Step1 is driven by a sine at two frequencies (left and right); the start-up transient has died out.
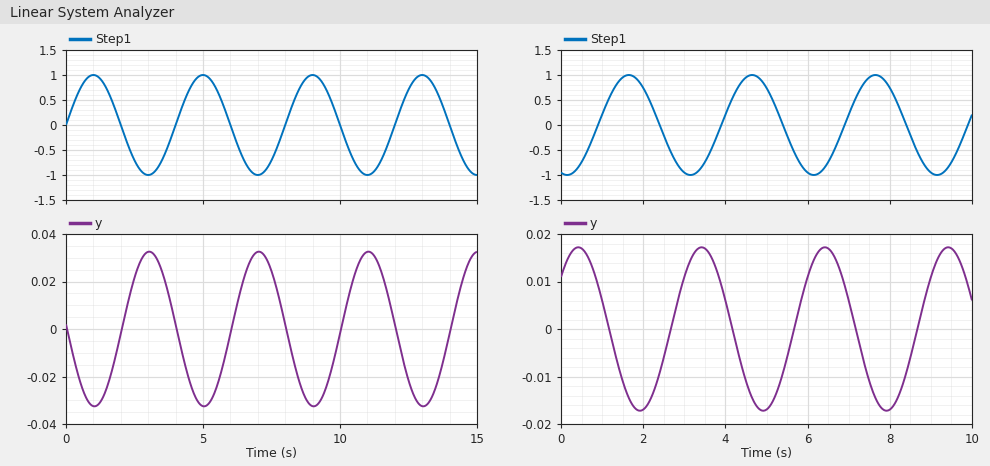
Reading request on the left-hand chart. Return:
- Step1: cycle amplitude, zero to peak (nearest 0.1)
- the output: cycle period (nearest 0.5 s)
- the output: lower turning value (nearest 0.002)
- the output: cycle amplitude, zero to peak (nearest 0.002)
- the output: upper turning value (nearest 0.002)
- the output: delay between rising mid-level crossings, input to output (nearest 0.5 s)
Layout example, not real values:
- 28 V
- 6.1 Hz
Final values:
- 1.0
- 4.0 s
- -0.032
- 0.032
- 0.032
- 2.0 s
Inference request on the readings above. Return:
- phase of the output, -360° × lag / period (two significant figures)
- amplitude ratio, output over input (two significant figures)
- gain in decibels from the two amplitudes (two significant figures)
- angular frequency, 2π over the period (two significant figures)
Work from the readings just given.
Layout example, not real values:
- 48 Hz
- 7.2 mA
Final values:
- -180°
- 0.032
- -30 dB
- 1.6 rad/s
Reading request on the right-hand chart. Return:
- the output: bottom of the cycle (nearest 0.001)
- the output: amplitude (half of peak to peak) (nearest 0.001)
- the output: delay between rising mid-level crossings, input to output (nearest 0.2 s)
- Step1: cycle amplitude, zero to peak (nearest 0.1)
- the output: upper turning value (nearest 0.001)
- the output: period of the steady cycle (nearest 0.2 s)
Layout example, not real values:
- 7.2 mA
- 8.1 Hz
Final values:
- -0.017
- 0.017
- 1.8 s
- 1.0
- 0.017
- 3.0 s
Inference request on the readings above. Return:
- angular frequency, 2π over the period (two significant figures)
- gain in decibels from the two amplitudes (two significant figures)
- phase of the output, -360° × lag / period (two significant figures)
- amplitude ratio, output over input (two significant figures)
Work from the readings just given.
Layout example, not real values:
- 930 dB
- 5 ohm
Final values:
- 2.1 rad/s
- -35 dB
- -220°
- 0.017
